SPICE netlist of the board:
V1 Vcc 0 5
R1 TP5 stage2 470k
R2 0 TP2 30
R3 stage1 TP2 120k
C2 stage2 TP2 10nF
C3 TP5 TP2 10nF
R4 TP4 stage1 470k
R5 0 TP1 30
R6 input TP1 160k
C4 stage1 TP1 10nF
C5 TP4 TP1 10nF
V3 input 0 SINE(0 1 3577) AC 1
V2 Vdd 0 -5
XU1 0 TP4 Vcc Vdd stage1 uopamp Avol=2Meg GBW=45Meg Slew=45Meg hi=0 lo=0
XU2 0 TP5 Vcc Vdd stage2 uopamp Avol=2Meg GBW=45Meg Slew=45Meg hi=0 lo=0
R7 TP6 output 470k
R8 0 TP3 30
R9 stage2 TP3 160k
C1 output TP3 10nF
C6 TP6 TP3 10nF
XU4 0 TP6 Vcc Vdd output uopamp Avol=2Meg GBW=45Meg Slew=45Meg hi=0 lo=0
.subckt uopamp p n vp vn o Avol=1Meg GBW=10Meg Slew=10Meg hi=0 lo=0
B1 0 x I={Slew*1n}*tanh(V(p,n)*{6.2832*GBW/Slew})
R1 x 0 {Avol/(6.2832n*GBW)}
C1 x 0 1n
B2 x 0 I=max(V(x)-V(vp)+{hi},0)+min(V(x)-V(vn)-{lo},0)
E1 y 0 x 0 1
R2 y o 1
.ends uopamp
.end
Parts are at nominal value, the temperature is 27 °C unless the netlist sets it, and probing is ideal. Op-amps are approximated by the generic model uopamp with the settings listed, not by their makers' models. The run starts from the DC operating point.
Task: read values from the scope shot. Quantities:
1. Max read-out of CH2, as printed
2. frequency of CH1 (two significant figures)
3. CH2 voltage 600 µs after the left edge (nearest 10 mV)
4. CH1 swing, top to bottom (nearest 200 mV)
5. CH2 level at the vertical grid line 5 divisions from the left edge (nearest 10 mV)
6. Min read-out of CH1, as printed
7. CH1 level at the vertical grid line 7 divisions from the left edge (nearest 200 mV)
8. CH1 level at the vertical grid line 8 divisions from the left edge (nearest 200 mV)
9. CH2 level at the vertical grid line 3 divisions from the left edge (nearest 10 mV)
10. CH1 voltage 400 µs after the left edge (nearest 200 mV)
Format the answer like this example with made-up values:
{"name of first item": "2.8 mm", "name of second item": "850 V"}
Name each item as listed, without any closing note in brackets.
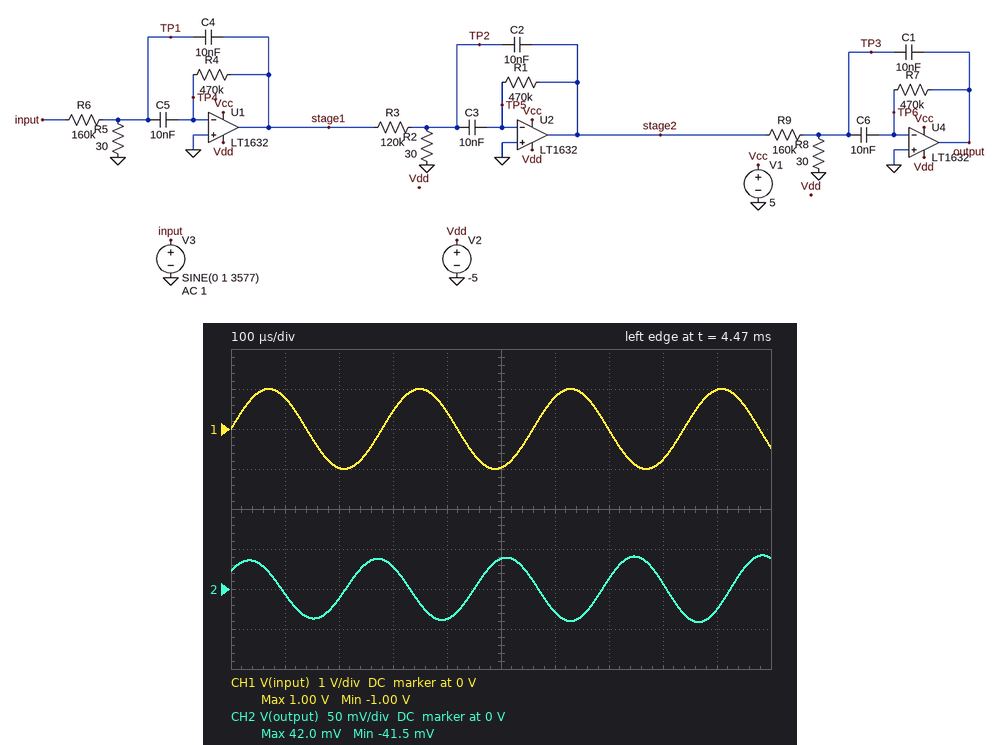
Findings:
{"Max read-out of CH2, as printed": "42.0 mV", "frequency of CH1": "3.6 kHz", "CH2 voltage 600 µs after the left edge": "-30 mV", "CH1 swing, top to bottom": "2.0 V", "CH2 level at the vertical grid line 5 divisions from the left edge": "40 mV", "Min read-out of CH1, as printed": "-1.00 V", "CH1 level at the vertical grid line 7 divisions from the left edge": "0 V", "CH1 level at the vertical grid line 8 divisions from the left edge": "-800 mV", "CH2 level at the vertical grid line 3 divisions from the left edge": "30 mV", "CH1 voltage 400 µs after the left edge": "400 mV"}
